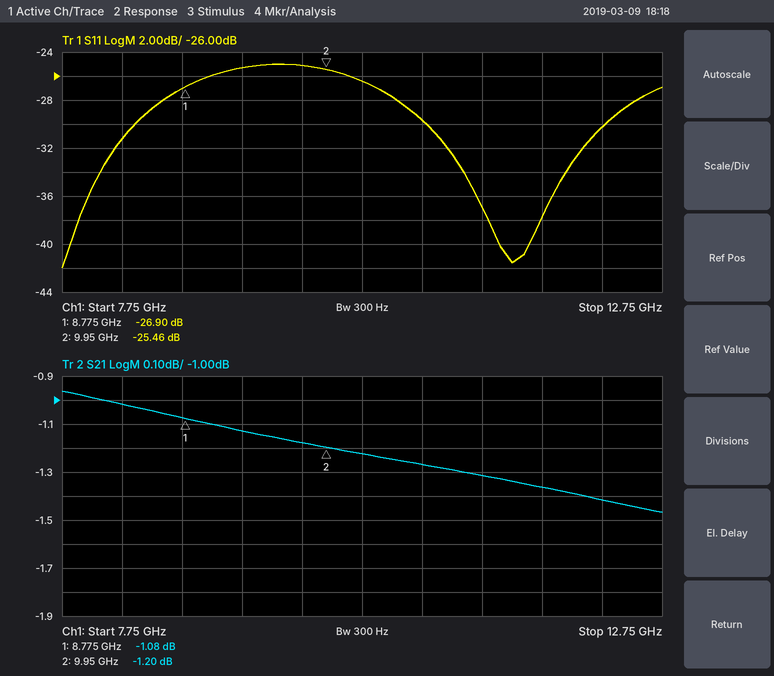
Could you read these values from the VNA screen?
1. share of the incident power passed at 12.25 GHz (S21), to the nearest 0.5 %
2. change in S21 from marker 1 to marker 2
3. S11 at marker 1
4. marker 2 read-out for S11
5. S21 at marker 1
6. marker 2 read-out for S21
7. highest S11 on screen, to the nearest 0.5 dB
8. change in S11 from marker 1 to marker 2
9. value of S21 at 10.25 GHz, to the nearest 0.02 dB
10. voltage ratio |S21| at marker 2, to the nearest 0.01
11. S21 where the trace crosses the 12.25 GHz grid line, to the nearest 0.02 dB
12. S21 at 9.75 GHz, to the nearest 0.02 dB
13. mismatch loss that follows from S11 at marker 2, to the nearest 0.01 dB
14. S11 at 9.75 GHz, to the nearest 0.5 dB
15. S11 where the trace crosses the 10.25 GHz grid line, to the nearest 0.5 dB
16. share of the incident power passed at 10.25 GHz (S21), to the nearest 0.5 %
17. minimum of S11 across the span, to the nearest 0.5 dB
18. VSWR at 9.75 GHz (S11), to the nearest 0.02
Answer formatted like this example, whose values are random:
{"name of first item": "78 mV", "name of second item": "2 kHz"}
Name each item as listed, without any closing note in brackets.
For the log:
{"share of the incident power passed at 12.25 GHz (S21), to the nearest 0.5 %": "72.0 %", "change in S21 from marker 1 to marker 2": "-0.12 dB", "S11 at marker 1": "-26.90 dB", "marker 2 read-out for S11": "-25.46 dB", "S21 at marker 1": "-1.08 dB", "marker 2 read-out for S21": "-1.20 dB", "highest S11 on screen, to the nearest 0.5 dB": "-25.0 dB", "change in S11 from marker 1 to marker 2": "1.44 dB", "value of S21 at 10.25 GHz, to the nearest 0.02 dB": "-1.22 dB", "voltage ratio |S21| at marker 2, to the nearest 0.01": "0.87", "S21 where the trace crosses the 12.25 GHz grid line, to the nearest 0.02 dB": "-1.42 dB", "S21 at 9.75 GHz, to the nearest 0.02 dB": "-1.18 dB", "mismatch loss that follows from S11 at marker 2, to the nearest 0.01 dB": "0.01 dB", "S11 at 9.75 GHz, to the nearest 0.5 dB": "-25.0 dB", "S11 where the trace crosses the 10.25 GHz grid line, to the nearest 0.5 dB": "-26.5 dB", "share of the incident power passed at 10.25 GHz (S21), to the nearest 0.5 %": "75.5 %", "minimum of S11 across the span, to the nearest 0.5 dB": "-42.0 dB", "VSWR at 9.75 GHz (S11), to the nearest 0.02": "1.12"}
